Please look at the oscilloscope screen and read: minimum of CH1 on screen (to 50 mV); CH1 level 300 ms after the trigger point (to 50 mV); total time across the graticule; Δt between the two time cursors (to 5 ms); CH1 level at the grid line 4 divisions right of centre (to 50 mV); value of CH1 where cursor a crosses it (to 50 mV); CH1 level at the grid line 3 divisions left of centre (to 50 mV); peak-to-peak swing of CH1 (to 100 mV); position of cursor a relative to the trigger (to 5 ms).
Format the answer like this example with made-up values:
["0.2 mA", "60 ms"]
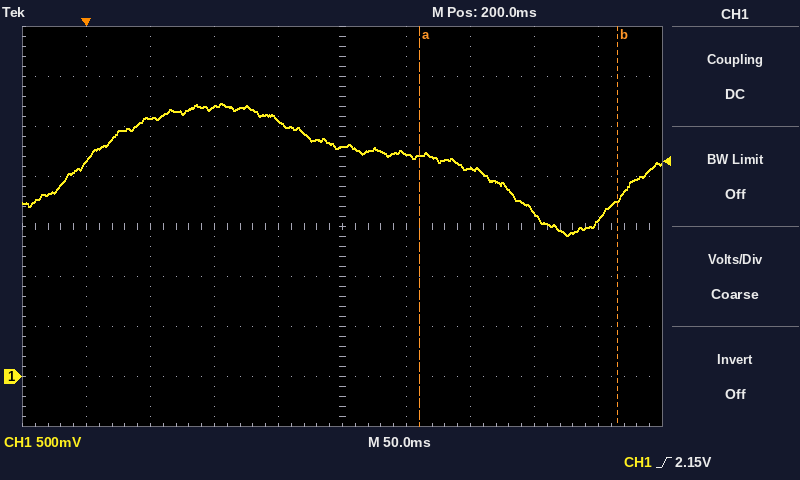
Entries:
["1.40 V", "2.10 V", "500 ms", "155 ms", "1.55 V", "2.20 V", "2.60 V", "1.30 V", "+260 ms"]
